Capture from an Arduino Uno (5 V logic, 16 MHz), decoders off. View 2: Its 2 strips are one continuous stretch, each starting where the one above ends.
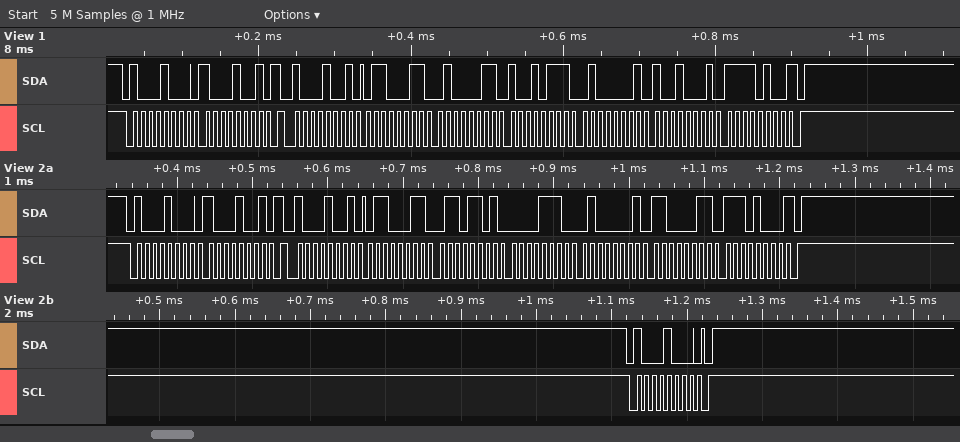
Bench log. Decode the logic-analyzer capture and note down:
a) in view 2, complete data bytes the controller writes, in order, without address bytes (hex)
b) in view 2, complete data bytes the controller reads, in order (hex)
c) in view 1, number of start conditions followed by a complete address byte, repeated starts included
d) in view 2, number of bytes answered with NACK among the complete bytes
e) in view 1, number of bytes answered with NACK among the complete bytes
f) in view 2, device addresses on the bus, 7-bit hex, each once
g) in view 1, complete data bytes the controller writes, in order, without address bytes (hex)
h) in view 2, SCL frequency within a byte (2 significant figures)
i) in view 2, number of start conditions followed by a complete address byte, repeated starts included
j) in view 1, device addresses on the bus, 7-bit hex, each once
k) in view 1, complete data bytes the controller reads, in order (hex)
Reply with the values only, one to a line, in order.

89
63 6D 0E 41 C3 E8
2
1
1
0x44
89
100 kHz
3
0x44
63 43 97 41 91 F4
